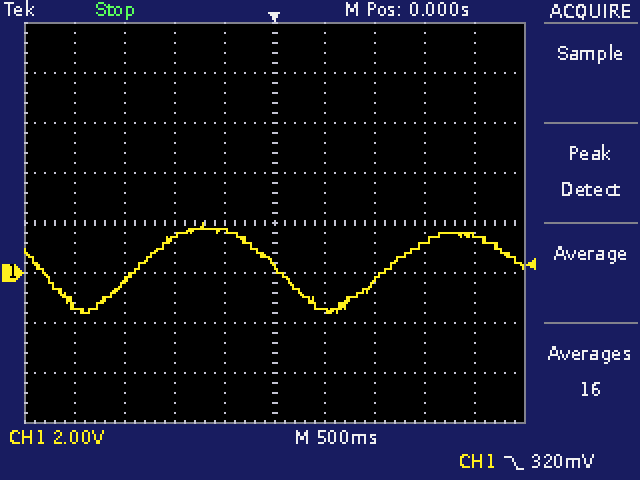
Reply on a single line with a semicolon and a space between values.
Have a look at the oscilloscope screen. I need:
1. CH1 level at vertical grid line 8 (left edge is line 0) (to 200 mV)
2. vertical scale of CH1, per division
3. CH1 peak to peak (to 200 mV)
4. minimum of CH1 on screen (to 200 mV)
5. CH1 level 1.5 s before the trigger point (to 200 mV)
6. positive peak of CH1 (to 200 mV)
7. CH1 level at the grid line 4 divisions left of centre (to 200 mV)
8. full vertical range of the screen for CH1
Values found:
1.2 V; 2 V; 3.6 V; -1.6 V; -400 mV; 2.0 V; -1.2 V; 16 V
